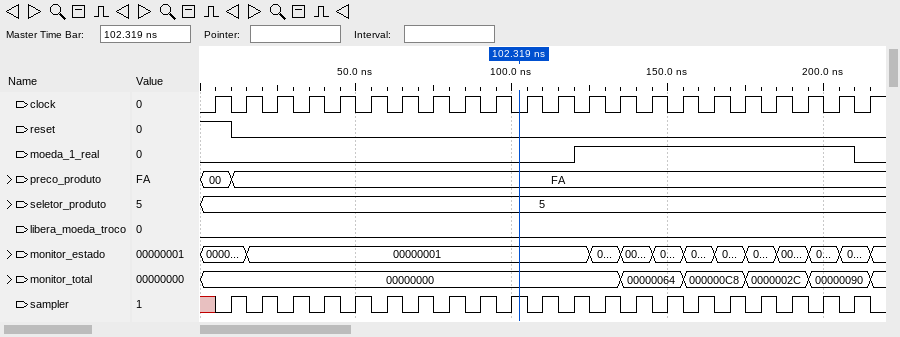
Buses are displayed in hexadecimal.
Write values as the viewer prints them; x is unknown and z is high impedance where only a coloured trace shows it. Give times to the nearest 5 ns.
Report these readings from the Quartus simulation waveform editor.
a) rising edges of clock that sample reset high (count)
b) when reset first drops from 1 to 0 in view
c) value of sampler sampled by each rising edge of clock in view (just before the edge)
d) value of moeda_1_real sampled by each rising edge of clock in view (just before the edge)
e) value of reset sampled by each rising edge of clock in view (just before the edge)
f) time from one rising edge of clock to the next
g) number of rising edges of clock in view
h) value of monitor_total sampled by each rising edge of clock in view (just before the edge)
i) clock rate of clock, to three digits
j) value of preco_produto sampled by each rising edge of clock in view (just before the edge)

1
10 ns
x 1 1 1 1 1 1 1 1 1 1 1 1 1 1 1 1 1 1 1 1 1
0 0 0 0 0 0 0 0 0 0 0 0 1 1 1 1 1 1 1 1 1 0
1 0 0 0 0 0 0 0 0 0 0 0 0 0 0 0 0 0 0 0 0 0
10 ns
22
00000000, 00000000, 00000000, 00000000, 00000000, 00000000, 00000000, 00000000, 00000000, 00000000, 00000000, 00000000, 00000000, 00000000, 00000064, 00000064, 000000C8, 000000C8, 0000002C, 0000002C, 00000090, 00000090
100 MHz
00, FA, FA, FA, FA, FA, FA, FA, FA, FA, FA, FA, FA, FA, FA, FA, FA, FA, FA, FA, FA, FA
